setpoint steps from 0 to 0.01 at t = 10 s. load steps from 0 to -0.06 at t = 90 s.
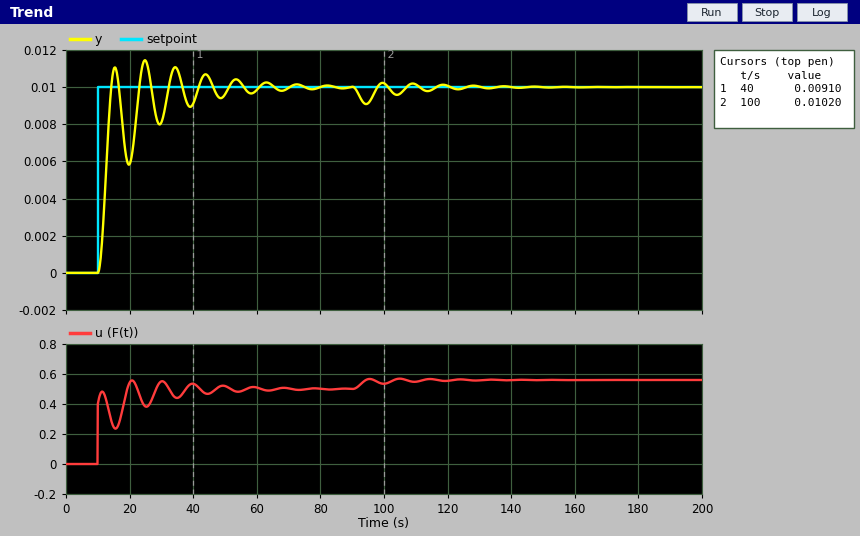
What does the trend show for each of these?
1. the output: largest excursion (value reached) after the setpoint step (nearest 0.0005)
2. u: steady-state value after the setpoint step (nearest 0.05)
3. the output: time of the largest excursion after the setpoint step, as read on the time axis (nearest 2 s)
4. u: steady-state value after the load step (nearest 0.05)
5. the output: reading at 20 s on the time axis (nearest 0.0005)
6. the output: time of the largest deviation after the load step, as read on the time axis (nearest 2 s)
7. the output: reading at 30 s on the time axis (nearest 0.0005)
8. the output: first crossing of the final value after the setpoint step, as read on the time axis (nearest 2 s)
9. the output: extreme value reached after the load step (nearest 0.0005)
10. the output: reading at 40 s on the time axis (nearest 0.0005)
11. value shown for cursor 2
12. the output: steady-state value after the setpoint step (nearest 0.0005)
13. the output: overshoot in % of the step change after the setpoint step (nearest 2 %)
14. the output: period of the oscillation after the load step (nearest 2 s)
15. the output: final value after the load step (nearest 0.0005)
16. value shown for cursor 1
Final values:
0.0115
0.50
24 s
0.55
0.0060
94 s
0.0080
14 s
0.0090
0.0090
0.01020
0.0100
14 %
10 s
0.0100
0.00910
